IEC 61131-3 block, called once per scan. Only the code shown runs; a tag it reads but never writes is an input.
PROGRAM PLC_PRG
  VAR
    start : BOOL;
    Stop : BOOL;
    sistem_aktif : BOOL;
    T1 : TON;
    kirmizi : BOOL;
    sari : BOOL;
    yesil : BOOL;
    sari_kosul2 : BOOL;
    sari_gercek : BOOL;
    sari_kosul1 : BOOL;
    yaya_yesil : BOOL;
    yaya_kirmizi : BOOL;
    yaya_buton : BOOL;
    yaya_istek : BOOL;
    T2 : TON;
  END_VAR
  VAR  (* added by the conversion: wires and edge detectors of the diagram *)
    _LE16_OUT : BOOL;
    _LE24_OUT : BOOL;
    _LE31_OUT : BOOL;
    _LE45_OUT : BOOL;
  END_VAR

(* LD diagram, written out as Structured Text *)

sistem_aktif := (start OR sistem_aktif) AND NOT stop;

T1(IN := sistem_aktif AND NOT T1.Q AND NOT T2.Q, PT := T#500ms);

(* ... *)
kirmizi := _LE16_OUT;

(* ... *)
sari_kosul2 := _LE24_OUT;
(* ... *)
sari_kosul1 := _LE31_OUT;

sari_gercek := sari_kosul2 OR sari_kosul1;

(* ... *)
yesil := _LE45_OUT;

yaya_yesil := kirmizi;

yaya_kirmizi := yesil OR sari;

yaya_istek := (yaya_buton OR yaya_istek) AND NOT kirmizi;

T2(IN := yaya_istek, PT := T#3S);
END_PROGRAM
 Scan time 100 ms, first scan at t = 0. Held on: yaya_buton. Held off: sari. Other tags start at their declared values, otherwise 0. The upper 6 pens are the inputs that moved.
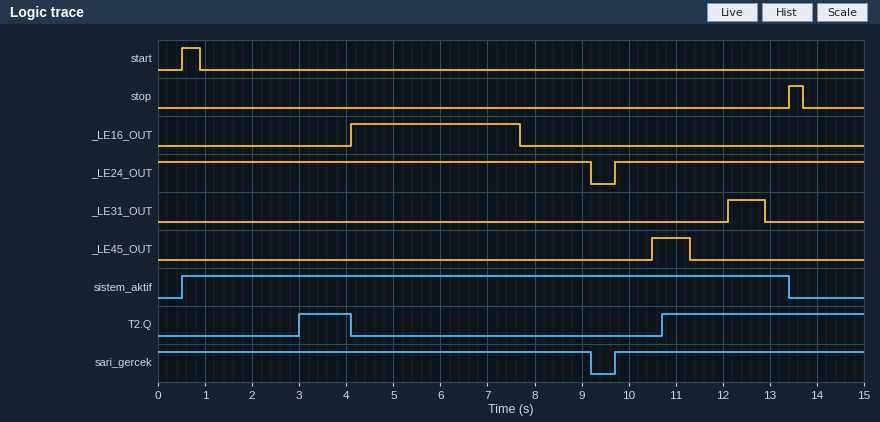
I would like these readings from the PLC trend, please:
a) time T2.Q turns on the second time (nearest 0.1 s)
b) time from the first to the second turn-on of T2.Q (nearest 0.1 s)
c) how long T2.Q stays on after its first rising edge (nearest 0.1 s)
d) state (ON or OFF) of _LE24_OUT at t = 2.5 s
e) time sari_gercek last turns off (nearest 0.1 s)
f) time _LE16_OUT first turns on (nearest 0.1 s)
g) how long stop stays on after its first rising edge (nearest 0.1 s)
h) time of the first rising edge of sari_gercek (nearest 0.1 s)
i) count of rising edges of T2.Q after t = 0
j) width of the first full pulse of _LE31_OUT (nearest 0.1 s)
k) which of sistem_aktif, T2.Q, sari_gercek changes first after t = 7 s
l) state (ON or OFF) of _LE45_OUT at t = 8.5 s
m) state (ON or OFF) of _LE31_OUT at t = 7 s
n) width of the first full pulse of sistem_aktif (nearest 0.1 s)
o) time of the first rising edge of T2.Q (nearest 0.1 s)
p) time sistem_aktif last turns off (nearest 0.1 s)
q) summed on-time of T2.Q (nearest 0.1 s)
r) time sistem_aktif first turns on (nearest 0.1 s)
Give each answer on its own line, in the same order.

10.7 s
7.7 s
1.1 s
ON
9.2 s
4.1 s
0.3 s
9.7 s
2
0.8 s
sari_gercek
OFF
OFF
12.9 s
3.0 s
13.4 s
5.4 s
0.5 s
